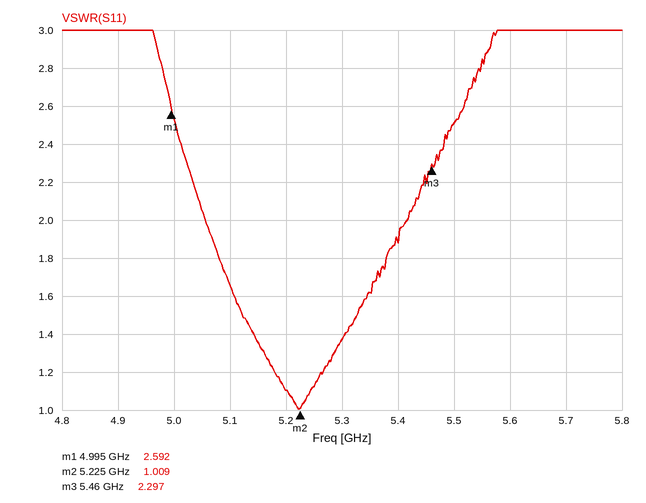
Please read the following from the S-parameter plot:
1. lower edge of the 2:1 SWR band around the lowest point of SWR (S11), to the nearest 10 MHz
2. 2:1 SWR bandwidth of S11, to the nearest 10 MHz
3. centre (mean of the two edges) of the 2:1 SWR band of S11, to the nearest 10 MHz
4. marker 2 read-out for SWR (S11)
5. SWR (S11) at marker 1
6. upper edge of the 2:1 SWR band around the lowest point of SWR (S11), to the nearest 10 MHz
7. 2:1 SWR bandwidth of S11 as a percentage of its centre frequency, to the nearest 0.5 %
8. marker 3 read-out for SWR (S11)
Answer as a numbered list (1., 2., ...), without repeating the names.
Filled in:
1. 5.06 GHz
2. 360 MHz
3. 5.24 GHz
4. 1.009
5. 2.592
6. 5.42 GHz
7. 7.0 %
8. 2.297
